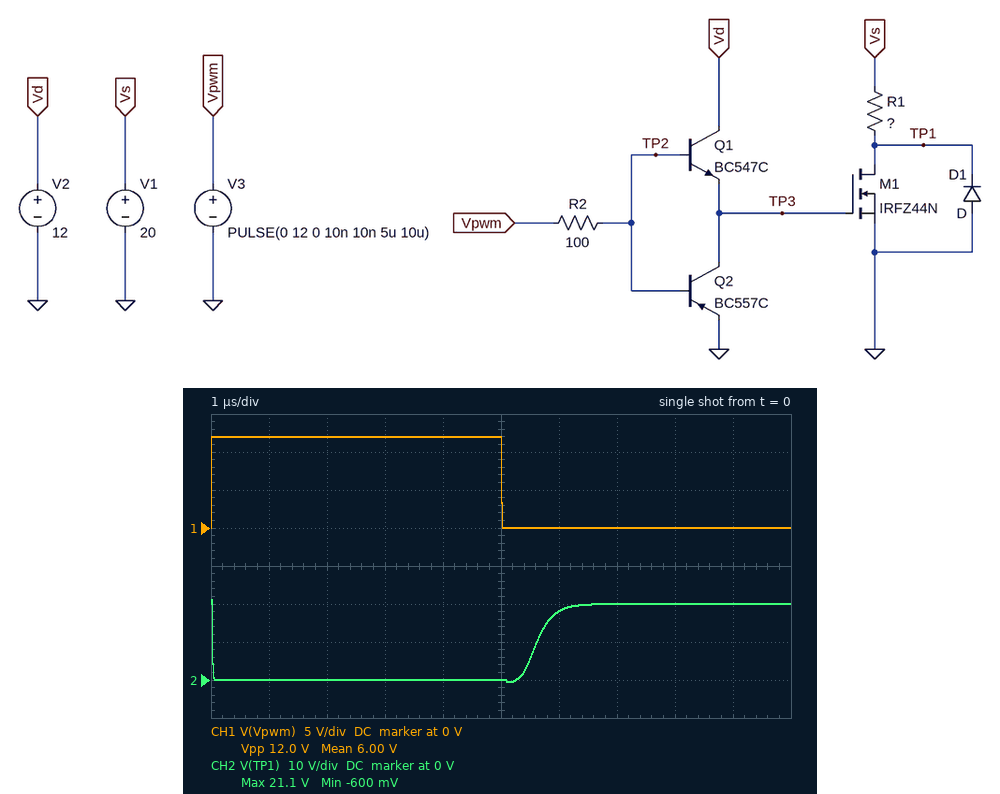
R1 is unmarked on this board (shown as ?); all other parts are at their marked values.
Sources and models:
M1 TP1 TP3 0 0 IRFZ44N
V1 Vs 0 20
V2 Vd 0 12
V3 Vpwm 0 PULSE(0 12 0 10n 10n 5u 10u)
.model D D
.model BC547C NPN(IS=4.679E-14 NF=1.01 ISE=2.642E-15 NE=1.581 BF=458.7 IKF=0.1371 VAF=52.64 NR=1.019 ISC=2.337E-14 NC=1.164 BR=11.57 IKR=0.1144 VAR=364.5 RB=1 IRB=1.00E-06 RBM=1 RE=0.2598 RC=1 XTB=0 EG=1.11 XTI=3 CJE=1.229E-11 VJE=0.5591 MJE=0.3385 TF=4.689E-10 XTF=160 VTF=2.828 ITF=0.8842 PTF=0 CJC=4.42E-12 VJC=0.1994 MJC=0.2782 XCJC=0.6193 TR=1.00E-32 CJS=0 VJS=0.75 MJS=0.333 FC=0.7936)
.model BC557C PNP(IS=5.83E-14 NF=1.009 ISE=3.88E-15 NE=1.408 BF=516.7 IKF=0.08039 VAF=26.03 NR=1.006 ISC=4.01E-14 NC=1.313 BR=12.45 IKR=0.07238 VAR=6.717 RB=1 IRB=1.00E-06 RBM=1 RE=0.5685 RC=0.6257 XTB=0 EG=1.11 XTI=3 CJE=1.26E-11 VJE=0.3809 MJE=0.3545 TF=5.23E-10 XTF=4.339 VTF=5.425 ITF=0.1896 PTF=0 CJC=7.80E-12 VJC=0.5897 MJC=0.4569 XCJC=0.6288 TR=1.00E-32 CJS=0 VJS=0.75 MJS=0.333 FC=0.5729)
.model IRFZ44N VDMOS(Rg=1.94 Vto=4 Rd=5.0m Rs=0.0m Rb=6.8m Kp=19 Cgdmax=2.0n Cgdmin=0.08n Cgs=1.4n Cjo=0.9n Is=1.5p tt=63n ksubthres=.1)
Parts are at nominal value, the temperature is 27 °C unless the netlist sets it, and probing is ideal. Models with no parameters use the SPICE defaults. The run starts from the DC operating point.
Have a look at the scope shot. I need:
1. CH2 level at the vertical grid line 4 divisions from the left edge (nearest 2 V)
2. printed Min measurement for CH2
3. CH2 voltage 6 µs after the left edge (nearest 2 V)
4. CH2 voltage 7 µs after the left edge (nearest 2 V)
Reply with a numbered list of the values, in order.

1. 0 V
2. -600 mV
3. 18 V
4. 20 V
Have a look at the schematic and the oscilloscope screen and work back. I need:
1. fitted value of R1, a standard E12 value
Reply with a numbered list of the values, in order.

1. 680 Ω
